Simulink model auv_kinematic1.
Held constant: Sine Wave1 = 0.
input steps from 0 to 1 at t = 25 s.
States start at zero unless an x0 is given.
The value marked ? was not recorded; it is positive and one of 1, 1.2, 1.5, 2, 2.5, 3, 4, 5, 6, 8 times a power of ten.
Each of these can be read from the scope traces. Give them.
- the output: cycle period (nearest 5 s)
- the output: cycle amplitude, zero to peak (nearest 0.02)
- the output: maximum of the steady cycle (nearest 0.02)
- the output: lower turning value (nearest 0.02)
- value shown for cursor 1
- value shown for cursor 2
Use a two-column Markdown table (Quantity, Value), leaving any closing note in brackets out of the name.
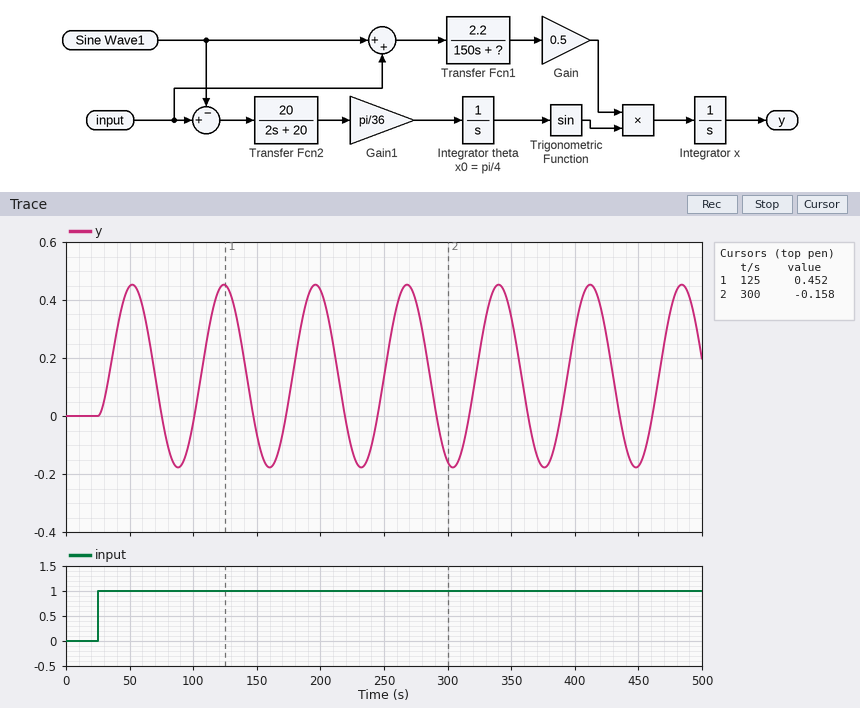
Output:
| Quantity | Value |
|---|---|
| the output: cycle period | 70 s |
| the output: cycle amplitude, zero to peak | 0.32 |
| the output: maximum of the steady cycle | 0.46 |
| the output: lower turning value | -0.18 |
| value shown for cursor 1 | 0.452 |
| value shown for cursor 2 | -0.158 |
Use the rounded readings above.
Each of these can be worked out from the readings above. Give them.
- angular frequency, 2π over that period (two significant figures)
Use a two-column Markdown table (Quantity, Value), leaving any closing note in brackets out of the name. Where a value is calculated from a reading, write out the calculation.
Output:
| Quantity | Value |
|---|---|
| angular frequency, 2π over that period | 2π / 70 = 0.090 rad/s |
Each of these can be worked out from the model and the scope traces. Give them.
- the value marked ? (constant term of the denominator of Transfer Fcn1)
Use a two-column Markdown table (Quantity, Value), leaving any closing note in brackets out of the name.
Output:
| Quantity | Value |
|---|---|
| the value marked ? | 40 |
